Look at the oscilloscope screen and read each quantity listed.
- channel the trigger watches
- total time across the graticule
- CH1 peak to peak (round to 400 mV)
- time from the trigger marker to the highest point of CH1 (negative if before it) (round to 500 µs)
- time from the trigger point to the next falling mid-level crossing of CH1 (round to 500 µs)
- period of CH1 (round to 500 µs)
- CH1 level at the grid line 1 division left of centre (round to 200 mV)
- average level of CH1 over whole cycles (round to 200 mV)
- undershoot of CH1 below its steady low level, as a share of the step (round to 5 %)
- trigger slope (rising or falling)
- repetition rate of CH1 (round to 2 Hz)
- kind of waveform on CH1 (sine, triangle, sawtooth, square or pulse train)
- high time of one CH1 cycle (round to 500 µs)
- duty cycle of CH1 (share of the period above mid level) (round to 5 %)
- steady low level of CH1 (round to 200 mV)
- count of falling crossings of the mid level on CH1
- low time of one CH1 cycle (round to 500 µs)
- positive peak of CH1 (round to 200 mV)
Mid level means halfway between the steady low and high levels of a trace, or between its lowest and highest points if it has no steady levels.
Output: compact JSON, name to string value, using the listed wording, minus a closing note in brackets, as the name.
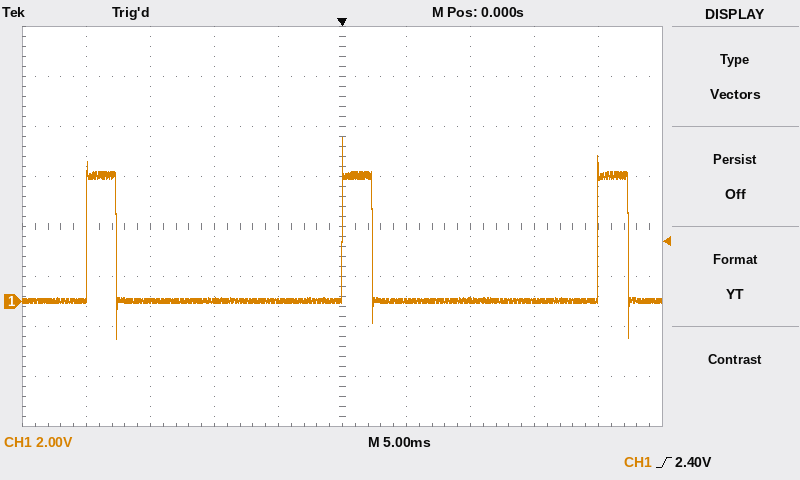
{"channel the trigger watches": "CH1", "total time across the graticule": "50 ms", "CH1 peak to peak": "8.0 V", "time from the trigger marker to the highest point of CH1 (negative if before it)": "0.0 ms", "time from the trigger point to the next falling mid-level crossing of CH1": "2.5 ms", "period of CH1": "20.0 ms", "CH1 level at the grid line 1 division left of centre": "0.0 V", "average level of CH1 over whole cycles": "600 mV", "undershoot of CH1 below its steady low level, as a share of the step": "30 %", "trigger slope": "rising", "repetition rate of CH1": "50 Hz", "kind of waveform on CH1": "pulse train", "high time of one CH1 cycle": "2.5 ms", "duty cycle of CH1 (share of the period above mid level)": "10 %", "steady low level of CH1": "0.0 V", "count of falling crossings of the mid level on CH1": "3", "low time of one CH1 cycle": "17.5 ms", "positive peak of CH1": "6.6 V"}
